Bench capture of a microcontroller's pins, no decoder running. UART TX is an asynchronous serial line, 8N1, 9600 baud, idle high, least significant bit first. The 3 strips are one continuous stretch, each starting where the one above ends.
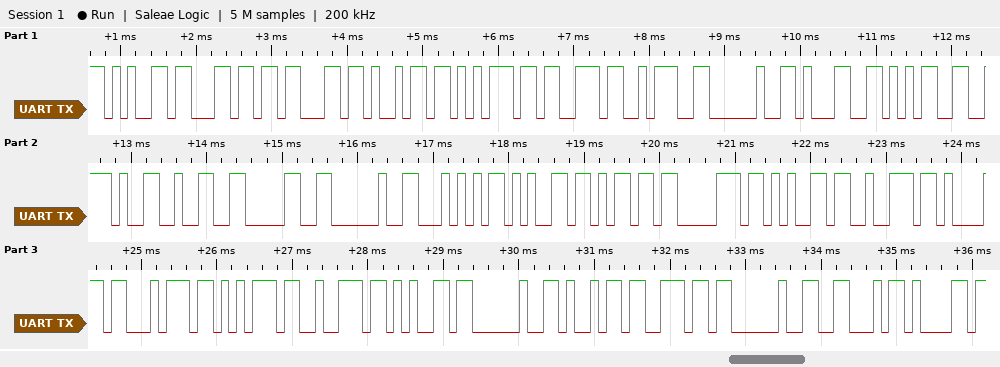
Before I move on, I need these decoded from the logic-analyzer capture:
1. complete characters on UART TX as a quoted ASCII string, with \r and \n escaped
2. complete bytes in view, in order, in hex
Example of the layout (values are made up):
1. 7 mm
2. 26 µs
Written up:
1. "elcius: 15.20 Temperature in Fa"
2. 0x65 0x6C 0x63 0x69 0x75 0x73 0x3A 0x20 0x31 0x35 0x2E 0x32 0x30 0x20 0x54 0x65 0x6D 0x70 0x65 0x72 0x61 0x74 0x75 0x72 0x65 0x20 0x69 0x6E 0x20 0x46 0x61
